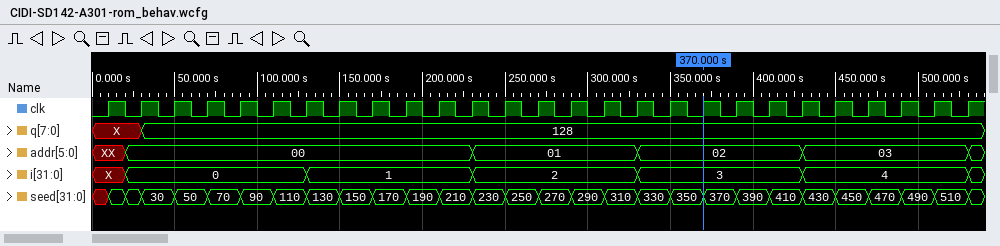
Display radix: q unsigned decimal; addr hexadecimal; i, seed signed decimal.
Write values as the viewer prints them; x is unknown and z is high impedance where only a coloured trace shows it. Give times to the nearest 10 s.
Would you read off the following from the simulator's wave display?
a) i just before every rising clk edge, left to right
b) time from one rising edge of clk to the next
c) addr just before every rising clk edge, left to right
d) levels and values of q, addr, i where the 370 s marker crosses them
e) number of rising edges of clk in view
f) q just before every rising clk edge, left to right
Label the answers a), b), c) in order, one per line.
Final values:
a) X, 0, 0, 0, 0, 0, 0, 1, 1, 1, 1, 1, 2, 2, 2, 2, 2, 3, 3, 3, 3, 3, 4, 4, 4, 4, 4
b) 20 s
c) XX, 00, 00, 00, 00, 00, 00, 00, 00, 00, 00, 00, 01, 01, 01, 01, 01, 02, 02, 02, 02, 02, 03, 03, 03, 03, 03
d) q=128, addr=02, i=3
e) 27
f) X, X, 128, 128, 128, 128, 128, 128, 128, 128, 128, 128, 128, 128, 128, 128, 128, 128, 128, 128, 128, 128, 128, 128, 128, 128, 128
